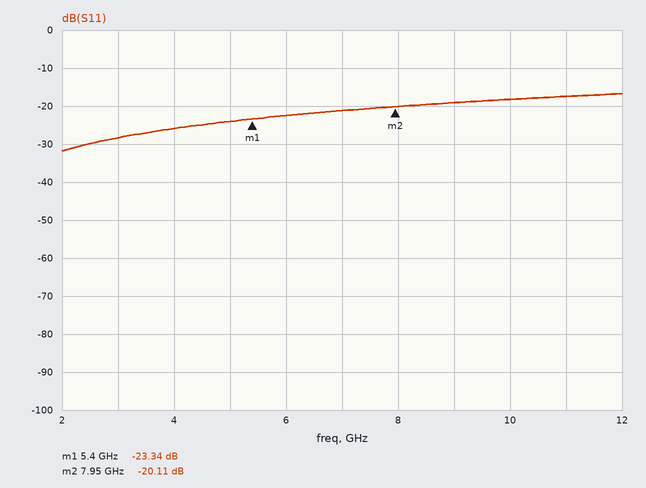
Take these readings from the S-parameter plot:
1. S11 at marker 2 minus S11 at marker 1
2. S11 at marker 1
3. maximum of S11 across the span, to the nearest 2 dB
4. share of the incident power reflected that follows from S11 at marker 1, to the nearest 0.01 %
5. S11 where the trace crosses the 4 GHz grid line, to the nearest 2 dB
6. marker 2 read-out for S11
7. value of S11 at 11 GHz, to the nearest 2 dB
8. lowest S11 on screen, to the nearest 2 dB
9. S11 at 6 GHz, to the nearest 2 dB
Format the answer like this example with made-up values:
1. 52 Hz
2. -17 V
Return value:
1. 3.23 dB
2. -23.34 dB
3. -16 dB
4. 0.46 %
5. -26 dB
6. -20.11 dB
7. -18 dB
8. -32 dB
9. -22 dB
